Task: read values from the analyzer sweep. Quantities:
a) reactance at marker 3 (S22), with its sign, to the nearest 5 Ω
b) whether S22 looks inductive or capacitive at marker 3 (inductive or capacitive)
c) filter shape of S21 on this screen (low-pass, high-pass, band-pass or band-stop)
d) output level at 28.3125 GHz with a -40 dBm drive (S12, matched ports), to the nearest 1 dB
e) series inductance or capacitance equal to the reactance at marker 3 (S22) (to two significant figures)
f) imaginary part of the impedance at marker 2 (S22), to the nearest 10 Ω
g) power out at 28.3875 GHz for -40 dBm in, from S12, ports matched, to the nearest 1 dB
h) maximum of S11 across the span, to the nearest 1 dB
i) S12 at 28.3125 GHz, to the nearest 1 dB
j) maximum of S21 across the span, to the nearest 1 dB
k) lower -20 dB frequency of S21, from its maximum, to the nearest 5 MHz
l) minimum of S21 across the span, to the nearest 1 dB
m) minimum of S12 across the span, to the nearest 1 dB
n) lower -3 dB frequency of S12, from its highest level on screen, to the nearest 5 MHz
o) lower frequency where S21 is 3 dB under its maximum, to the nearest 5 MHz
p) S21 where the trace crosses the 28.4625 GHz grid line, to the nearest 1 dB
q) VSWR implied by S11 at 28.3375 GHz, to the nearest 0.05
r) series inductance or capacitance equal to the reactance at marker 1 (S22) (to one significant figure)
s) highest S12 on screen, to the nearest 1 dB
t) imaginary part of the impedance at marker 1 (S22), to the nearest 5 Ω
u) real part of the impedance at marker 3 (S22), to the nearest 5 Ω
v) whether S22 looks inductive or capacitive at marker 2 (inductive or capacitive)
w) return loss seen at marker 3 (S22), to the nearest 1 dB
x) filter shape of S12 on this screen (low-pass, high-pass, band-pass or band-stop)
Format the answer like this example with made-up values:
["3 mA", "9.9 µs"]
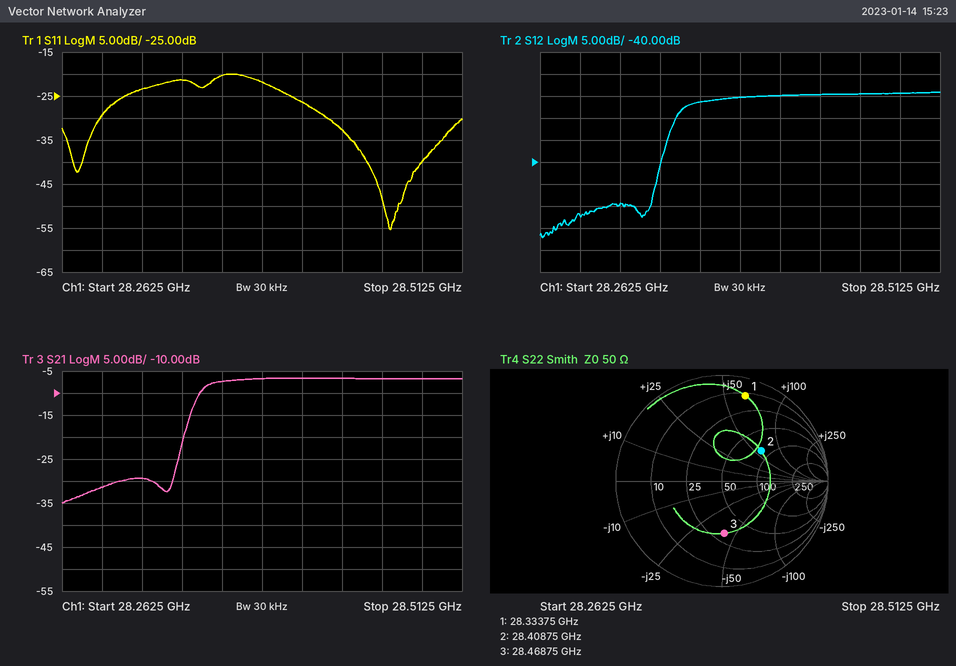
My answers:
["-40 Ω", "capacitive", "high-pass", "-90 dBm", "140 fF", "+60 Ω", "-65 dBm", "-20 dB", "-50 dB", "-7 dB", "28.335 GHz", "-35 dB", "-57 dB", "28.355 GHz", "28.350 GHz", "-7 dB", "1.20", "400 pH", "-24 dB", "+65 Ω", "30 Ω", "inductive", "6 dB", "high-pass"]
